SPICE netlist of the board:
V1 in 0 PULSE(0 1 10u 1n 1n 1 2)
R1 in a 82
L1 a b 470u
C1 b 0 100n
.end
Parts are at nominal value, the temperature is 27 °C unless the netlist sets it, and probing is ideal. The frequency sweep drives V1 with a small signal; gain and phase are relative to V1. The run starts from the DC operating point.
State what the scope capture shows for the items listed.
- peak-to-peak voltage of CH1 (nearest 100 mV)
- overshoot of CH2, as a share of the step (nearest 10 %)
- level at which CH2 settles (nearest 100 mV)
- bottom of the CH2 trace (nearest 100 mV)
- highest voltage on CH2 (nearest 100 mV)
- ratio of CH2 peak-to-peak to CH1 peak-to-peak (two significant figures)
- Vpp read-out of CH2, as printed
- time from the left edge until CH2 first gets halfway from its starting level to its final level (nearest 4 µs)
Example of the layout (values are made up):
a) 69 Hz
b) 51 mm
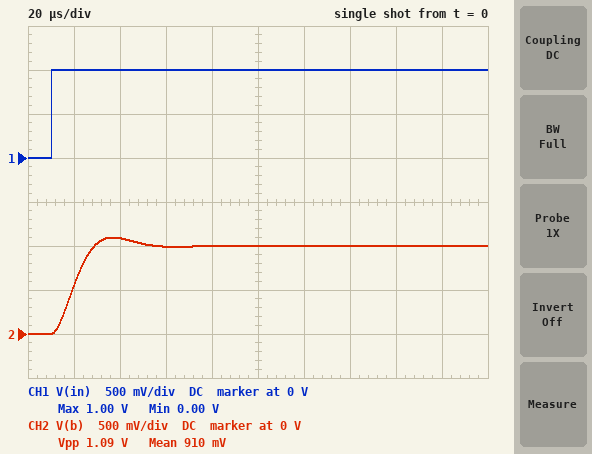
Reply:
a) 1.0 V
b) 10 %
c) 1.0 V
d) 0 V
e) 1.1 V
f) 1.1
g) 1.09 V
h) 20 µs
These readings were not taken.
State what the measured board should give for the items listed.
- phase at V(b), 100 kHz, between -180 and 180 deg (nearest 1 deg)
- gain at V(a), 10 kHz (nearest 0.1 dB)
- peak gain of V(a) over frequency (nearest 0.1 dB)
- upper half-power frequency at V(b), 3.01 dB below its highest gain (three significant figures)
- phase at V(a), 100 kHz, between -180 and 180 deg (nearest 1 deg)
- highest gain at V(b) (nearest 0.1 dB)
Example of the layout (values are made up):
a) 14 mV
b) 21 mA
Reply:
a) -164 deg
b) -1.5 dB
c) 0 dB
d) 25.9 kHz
e) 16 deg
f) 0.4 dB
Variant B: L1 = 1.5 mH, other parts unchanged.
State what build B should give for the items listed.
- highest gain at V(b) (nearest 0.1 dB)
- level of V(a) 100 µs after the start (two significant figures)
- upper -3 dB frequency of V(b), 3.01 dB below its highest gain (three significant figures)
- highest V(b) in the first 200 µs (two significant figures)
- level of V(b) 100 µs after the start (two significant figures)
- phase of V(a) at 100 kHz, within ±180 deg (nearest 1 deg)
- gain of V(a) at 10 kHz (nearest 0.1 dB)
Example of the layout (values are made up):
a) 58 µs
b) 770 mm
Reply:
a) 4.0 dB
b) 960 mV
c) 15.4 kHz
d) 1.3 V
e) 910 mV
f) 5 deg
g) -4.1 dB
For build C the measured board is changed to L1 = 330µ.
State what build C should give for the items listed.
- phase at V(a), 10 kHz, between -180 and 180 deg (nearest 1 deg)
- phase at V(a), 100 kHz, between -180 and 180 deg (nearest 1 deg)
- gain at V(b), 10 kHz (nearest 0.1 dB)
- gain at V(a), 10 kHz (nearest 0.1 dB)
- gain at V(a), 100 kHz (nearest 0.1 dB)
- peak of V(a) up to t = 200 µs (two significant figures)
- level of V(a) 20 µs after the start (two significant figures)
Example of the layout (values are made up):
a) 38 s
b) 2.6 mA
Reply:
a) -31 deg
b) 23 deg
c) -0.1 dB
d) -1.3 dB
e) -0.7 dB
f) 1.0 V
g) 450 mV
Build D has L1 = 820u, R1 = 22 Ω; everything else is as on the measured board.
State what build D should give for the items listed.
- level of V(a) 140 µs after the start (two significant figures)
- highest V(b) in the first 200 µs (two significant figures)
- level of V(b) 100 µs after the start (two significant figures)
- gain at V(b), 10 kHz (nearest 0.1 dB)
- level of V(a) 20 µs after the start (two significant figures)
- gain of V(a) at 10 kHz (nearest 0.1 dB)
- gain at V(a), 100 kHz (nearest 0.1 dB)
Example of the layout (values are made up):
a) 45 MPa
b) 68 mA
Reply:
a) 960 mV
b) 1.7 V
c) 1.3 V
d) 3.2 dB
e) 810 mV
f) -0.2 dB
g) 0 dB
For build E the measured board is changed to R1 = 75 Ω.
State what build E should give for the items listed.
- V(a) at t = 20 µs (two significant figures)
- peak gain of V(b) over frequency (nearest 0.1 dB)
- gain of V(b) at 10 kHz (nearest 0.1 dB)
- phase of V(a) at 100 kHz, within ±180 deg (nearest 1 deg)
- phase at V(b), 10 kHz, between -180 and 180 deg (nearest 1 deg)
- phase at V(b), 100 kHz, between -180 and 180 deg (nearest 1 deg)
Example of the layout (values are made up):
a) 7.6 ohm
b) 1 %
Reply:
a) 450 mV
b) 0.8 dB
c) 0.5 dB
d) 15 deg
e) -30 deg
f) -165 deg
